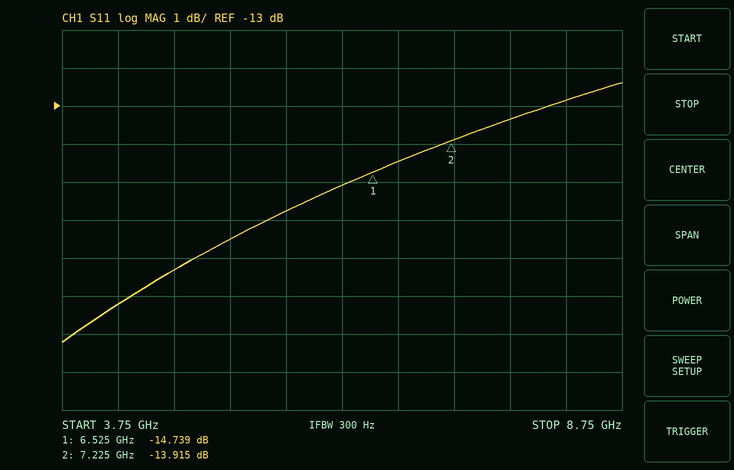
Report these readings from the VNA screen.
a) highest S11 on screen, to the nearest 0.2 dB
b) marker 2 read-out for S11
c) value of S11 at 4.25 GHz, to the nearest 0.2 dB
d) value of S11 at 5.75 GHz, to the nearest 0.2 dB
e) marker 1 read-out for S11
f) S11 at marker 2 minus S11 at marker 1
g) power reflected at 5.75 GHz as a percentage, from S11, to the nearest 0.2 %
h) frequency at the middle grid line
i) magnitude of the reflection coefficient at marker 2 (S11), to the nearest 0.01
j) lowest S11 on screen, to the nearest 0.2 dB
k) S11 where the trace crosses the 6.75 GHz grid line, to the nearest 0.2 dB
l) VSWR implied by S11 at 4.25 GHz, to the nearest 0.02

-12.4 dB
-13.915 dB
-18.2 dB
-15.8 dB
-14.739 dB
0.824 dB
2.6 %
6.25 GHz
0.20
-19.2 dB
-14.4 dB
1.28
